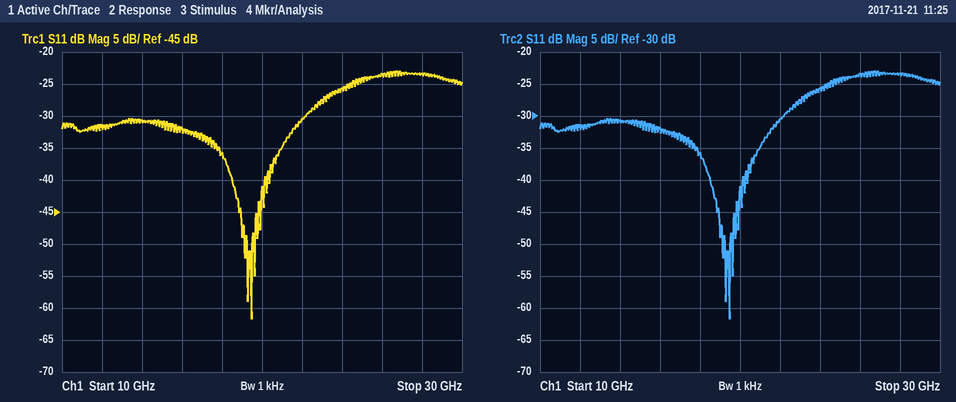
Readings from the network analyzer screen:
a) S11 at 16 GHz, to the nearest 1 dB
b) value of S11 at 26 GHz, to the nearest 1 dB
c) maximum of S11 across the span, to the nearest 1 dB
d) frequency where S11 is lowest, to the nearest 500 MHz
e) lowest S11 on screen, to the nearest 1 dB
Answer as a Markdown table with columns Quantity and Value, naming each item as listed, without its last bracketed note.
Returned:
| Quantity | Value |
|---|---|
| S11 at 16 GHz, to the nearest 1 dB | -32 dB |
| value of S11 at 26 GHz, to the nearest 1 dB | -23 dB |
| maximum of S11 across the span, to the nearest 1 dB | -23 dB |
| frequency where S11 is lowest, to the nearest 500 MHz | 19.5 GHz |
| lowest S11 on screen, to the nearest 1 dB | -62 dB |
